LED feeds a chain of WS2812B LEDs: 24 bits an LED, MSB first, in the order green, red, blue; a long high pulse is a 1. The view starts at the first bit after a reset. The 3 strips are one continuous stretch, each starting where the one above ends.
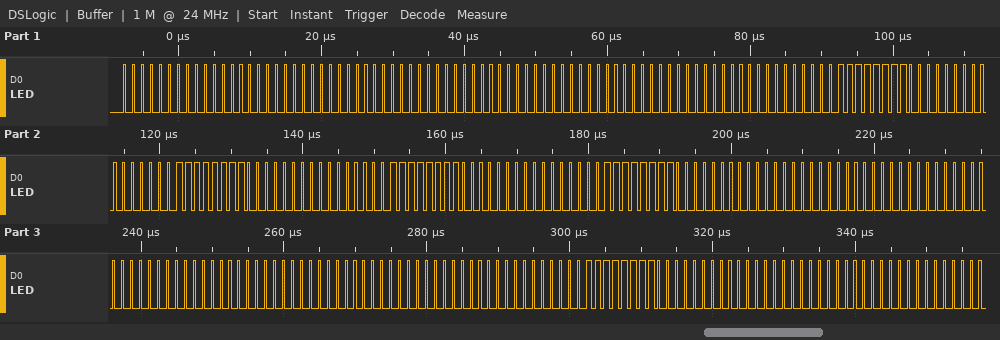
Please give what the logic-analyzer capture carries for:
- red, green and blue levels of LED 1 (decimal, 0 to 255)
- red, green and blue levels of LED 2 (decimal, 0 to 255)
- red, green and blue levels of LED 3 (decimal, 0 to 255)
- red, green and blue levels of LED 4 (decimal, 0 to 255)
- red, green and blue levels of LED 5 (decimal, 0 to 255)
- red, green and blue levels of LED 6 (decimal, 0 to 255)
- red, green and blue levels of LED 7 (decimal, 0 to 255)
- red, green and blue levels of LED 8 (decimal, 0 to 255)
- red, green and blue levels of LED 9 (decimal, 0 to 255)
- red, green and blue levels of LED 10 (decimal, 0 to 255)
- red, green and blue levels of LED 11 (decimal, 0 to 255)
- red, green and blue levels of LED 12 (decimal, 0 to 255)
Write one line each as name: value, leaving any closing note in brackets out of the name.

red, green and blue levels of LED 1: 0, 0, 0
red, green and blue levels of LED 2: 0, 0, 0
red, green and blue levels of LED 3: 0, 0, 0
red, green and blue levels of LED 4: 255, 0, 0
red, green and blue levels of LED 5: 255, 0, 0
red, green and blue levels of LED 6: 255, 0, 0
red, green and blue levels of LED 7: 255, 0, 0
red, green and blue levels of LED 8: 0, 0, 0
red, green and blue levels of LED 9: 0, 0, 0
red, green and blue levels of LED 10: 0, 0, 0
red, green and blue levels of LED 11: 255, 0, 0
red, green and blue levels of LED 12: 0, 0, 0
